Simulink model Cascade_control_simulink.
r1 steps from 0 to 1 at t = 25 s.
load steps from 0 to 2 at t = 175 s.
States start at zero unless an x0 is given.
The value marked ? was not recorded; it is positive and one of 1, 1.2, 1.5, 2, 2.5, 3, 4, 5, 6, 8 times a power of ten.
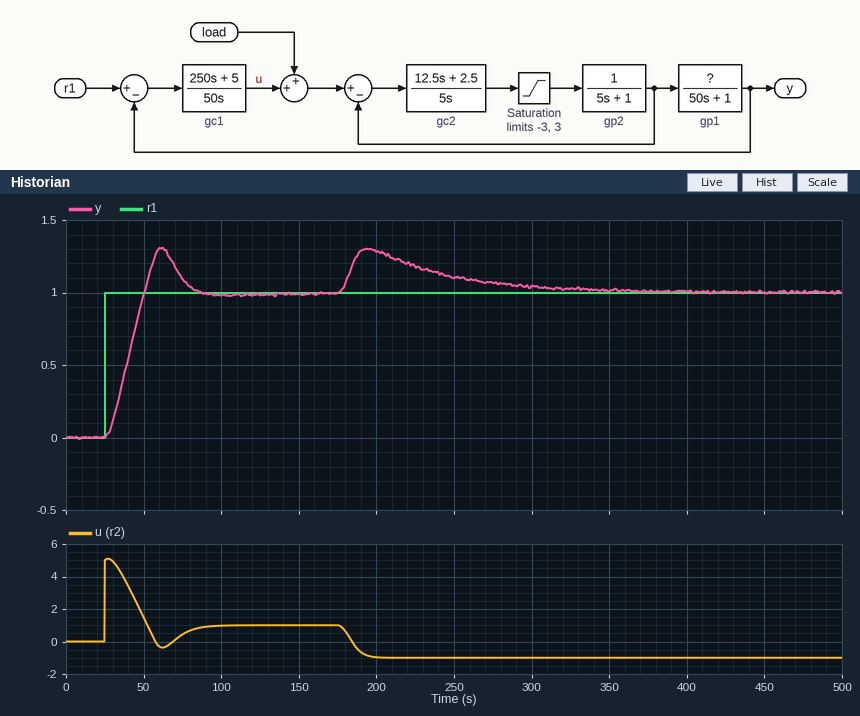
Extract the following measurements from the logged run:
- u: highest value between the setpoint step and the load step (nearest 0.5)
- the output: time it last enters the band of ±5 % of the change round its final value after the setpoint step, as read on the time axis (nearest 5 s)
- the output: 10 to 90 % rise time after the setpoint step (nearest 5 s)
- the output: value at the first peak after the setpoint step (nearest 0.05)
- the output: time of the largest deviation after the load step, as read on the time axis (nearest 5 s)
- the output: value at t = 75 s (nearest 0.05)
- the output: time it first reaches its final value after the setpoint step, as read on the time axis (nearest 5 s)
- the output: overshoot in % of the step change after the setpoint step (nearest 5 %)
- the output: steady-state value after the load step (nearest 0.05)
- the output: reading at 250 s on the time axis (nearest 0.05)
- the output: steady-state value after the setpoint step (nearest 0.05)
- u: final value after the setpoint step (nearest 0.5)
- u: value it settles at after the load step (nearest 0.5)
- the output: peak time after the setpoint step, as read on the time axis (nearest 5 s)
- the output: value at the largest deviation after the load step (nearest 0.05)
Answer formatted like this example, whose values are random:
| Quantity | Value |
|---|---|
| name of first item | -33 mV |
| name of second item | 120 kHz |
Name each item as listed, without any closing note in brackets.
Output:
| Quantity | Value |
|---|---|
| u: highest value between the setpoint step and the load step | 5.0 |
| the output: time it last enters the band of ±5 % of the change round its final value after the setpoint step, as read on the time axis | 80 s |
| the output: 10 to 90 % rise time after the setpoint step | 20 s |
| the output: value at the first peak after the setpoint step | 1.30 |
| the output: time of the largest deviation after the load step, as read on the time axis | 195 s |
| the output: value at t = 75 s | 1.10 |
| the output: time it first reaches its final value after the setpoint step, as read on the time axis | 50 s |
| the output: overshoot in % of the step change after the setpoint step | 30 % |
| the output: steady-state value after the load step | 1.00 |
| the output: reading at 250 s on the time axis | 1.10 |
| the output: steady-state value after the setpoint step | 1.00 |
| u: final value after the setpoint step | 1.0 |
| u: value it settles at after the load step | -1.0 |
| the output: peak time after the setpoint step, as read on the time axis | 60 s |
| the output: value at the largest deviation after the load step | 1.30 |
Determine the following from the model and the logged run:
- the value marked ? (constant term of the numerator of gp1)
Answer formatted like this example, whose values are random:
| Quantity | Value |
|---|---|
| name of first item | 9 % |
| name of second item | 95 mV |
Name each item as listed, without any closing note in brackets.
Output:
| Quantity | Value |
|---|---|
| the value marked ? | 1 |
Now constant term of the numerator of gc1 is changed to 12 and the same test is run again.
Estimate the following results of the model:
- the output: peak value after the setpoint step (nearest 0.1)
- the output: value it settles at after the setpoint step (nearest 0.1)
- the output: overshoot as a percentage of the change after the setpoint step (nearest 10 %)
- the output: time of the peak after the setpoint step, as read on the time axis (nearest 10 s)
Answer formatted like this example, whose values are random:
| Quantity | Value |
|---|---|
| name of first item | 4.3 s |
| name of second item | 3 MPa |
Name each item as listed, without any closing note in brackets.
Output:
| Quantity | Value |
|---|---|
| the output: peak value after the setpoint step | 1.7 |
| the output: value it settles at after the setpoint step | 1.0 |
| the output: overshoot as a percentage of the change after the setpoint step | 70 % |
| the output: time of the peak after the setpoint step, as read on the time axis | 70 s |
